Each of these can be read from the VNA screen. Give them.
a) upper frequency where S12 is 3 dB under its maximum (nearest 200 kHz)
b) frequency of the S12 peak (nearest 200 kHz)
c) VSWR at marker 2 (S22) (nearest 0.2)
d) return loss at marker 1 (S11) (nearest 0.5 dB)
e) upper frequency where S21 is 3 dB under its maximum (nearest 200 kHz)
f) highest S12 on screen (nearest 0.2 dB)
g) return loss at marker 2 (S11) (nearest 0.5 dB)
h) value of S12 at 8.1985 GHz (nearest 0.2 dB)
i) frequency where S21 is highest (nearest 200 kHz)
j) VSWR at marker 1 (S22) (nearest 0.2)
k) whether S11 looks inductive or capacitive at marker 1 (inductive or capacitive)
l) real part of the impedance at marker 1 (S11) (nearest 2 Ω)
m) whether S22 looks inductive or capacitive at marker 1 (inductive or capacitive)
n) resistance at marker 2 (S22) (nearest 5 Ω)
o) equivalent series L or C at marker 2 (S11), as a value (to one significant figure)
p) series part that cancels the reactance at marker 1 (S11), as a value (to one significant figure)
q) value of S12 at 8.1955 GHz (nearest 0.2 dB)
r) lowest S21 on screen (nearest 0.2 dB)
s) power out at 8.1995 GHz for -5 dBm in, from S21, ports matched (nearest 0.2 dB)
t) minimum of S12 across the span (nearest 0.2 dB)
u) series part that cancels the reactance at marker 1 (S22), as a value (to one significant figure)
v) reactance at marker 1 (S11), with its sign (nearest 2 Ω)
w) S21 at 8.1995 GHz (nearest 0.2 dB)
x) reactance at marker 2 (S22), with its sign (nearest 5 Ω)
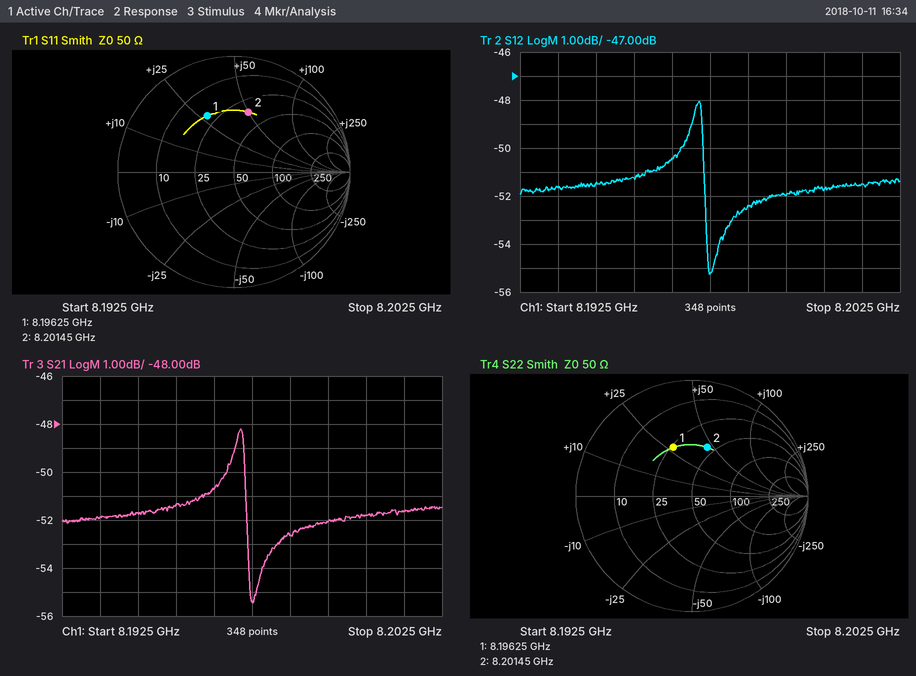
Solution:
8.1974 GHz
8.1972 GHz
2.6
5.5 dB
8.1974 GHz
-48.0 dB
5.5 dB
-52.4 dB
8.1972 GHz
2.6
inductive
20 Ω
inductive
45 Ω
1.0 nH
700 fF
-51.2 dB
-55.4 dB
-57.0 dBm
-55.2 dB
700 fF
+28 Ω
-52.0 dB
+45 Ω
